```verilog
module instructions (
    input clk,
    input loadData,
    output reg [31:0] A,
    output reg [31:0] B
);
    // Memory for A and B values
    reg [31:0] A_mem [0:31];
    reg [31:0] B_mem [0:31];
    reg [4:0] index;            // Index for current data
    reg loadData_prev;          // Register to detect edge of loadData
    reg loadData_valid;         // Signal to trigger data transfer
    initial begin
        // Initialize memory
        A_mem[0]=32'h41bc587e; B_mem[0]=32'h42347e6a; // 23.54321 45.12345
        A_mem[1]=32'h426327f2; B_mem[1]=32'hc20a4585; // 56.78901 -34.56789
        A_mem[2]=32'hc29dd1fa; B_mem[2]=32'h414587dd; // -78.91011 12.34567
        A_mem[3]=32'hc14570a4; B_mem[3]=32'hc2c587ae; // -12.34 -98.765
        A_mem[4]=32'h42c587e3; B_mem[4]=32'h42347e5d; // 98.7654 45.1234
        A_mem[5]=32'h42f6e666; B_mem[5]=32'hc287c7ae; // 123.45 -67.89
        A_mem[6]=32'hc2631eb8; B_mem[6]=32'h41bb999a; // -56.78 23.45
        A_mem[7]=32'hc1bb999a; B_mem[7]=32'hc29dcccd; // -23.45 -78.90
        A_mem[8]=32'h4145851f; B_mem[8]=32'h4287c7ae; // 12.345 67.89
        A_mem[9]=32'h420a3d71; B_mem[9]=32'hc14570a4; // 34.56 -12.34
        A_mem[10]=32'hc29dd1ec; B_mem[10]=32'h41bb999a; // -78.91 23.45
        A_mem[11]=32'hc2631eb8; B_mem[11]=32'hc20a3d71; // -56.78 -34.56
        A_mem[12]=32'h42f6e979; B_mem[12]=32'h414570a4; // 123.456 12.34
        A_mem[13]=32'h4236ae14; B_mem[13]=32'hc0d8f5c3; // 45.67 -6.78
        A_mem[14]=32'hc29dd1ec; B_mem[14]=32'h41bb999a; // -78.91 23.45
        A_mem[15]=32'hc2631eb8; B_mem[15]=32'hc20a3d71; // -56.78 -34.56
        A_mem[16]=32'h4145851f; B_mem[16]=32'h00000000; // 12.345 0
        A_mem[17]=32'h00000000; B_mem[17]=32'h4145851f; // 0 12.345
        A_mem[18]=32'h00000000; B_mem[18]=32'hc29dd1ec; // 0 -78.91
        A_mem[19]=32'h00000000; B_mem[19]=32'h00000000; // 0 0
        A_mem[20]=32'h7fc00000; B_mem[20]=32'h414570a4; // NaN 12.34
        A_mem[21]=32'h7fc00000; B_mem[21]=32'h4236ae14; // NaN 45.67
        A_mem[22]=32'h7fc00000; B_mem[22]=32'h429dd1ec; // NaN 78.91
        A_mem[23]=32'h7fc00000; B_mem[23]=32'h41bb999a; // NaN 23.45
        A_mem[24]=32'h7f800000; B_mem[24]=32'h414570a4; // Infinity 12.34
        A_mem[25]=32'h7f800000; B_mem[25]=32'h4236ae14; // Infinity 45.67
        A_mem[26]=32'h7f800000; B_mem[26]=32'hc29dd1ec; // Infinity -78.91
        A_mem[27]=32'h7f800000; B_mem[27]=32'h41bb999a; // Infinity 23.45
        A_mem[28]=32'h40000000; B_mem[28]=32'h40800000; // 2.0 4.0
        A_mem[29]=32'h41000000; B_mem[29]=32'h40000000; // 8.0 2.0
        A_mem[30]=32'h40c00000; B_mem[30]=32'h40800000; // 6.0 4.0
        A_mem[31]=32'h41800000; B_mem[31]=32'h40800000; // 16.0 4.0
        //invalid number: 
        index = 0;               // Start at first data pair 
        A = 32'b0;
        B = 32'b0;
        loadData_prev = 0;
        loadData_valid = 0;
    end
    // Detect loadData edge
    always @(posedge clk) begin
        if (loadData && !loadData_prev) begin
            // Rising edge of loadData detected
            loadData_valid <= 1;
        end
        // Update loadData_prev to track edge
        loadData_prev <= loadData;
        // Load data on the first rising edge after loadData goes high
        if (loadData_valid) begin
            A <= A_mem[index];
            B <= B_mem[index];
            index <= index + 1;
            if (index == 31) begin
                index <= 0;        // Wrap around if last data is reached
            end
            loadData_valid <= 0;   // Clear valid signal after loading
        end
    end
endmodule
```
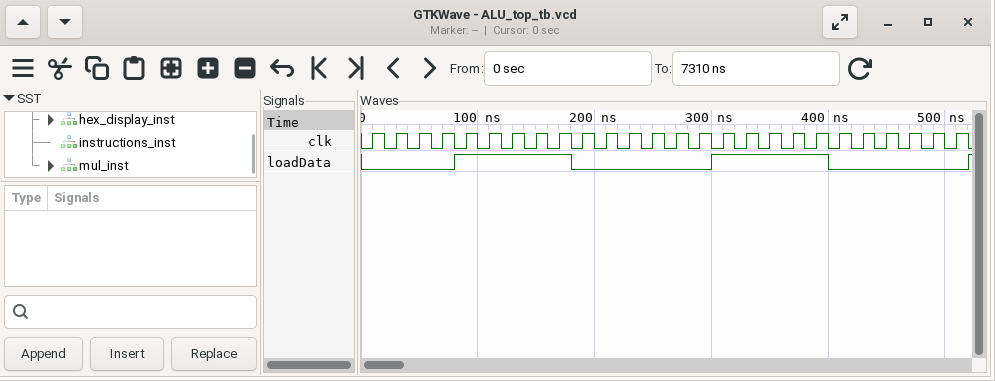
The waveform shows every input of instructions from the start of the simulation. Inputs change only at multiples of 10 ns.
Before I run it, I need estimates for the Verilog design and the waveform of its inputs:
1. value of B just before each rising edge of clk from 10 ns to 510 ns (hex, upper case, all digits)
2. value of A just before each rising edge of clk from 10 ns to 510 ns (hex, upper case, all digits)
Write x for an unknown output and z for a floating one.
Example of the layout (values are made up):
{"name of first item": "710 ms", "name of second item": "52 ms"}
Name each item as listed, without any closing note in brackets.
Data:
{"value of B just before each rising edge of clk from 10 ns to 510 ns": "00000000, 00000000, 00000000, 00000000, 00000000, 00000000, 42347E6A, 42347E6A, 42347E6A, 42347E6A, 42347E6A, 42347E6A, 42347E6A, 42347E6A, 42347E6A, 42347E6A, 42347E6A, C20A4585, C20A4585, C20A4585, C20A4585, C20A4585, C20A4585, C20A4585, C20A4585, C20A4585", "value of A just before each rising edge of clk from 10 ns to 510 ns": "00000000, 00000000, 00000000, 00000000, 00000000, 00000000, 41BC587E, 41BC587E, 41BC587E, 41BC587E, 41BC587E, 41BC587E, 41BC587E, 41BC587E, 41BC587E, 41BC587E, 41BC587E, 426327F2, 426327F2, 426327F2, 426327F2, 426327F2, 426327F2, 426327F2, 426327F2, 426327F2"}
